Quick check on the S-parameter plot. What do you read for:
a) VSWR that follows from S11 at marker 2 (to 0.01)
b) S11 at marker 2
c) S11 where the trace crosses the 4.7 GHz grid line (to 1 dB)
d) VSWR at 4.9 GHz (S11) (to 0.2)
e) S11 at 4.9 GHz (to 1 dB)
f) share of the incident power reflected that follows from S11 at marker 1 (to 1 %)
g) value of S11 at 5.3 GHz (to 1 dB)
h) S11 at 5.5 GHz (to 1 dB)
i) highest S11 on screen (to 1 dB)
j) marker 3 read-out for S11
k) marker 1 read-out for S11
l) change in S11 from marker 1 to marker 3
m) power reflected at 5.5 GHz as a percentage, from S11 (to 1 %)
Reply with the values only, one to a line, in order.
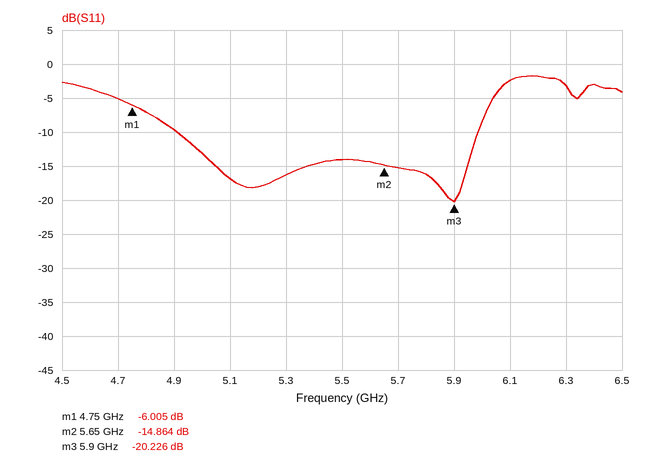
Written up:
1.44
-14.864 dB
-5 dB
2.0
-10 dB
25 %
-16 dB
-14 dB
-2 dB
-20.226 dB
-6.005 dB
-14.221 dB
4 %
